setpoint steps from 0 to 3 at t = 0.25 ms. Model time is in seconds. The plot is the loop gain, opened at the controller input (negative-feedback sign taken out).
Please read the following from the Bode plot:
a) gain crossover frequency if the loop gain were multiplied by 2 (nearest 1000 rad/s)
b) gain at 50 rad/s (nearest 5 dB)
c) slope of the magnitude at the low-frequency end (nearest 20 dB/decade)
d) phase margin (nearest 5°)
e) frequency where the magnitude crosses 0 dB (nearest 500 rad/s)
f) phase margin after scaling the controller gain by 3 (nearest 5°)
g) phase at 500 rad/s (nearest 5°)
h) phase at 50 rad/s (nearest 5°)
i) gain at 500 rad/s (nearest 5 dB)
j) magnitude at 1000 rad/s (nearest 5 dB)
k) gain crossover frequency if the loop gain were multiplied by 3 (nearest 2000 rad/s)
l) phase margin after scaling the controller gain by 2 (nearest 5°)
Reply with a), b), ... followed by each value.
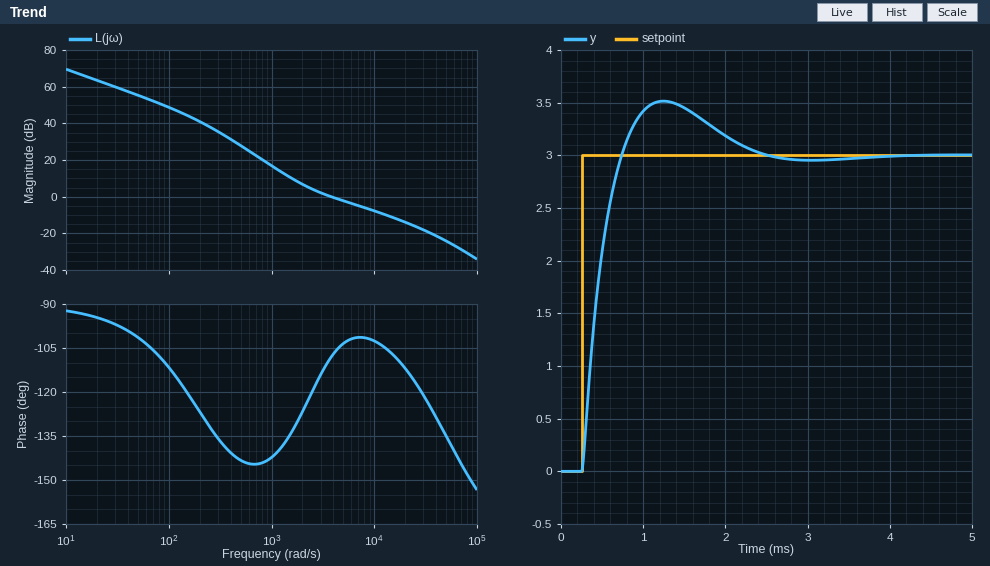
a) 8000 rad/s
b) 55 dB
c) -20 dB/decade
d) 70°
e) 4000 rad/s
f) 75°
g) -145°
h) -100°
i) 30 dB
j) 15 dB
k) 12000 rad/s
l) 80°
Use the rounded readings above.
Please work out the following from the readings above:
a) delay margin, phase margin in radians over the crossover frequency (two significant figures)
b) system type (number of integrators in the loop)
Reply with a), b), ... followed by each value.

a) 0.00031 s
b) 1
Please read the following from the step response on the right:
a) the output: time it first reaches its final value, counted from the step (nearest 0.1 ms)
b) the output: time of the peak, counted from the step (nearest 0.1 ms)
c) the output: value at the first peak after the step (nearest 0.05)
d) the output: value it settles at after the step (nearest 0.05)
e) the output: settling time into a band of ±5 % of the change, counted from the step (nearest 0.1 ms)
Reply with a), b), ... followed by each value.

a) 0.5 ms
b) 1.0 ms
c) 3.50
d) 3.00
e) 1.8 ms
